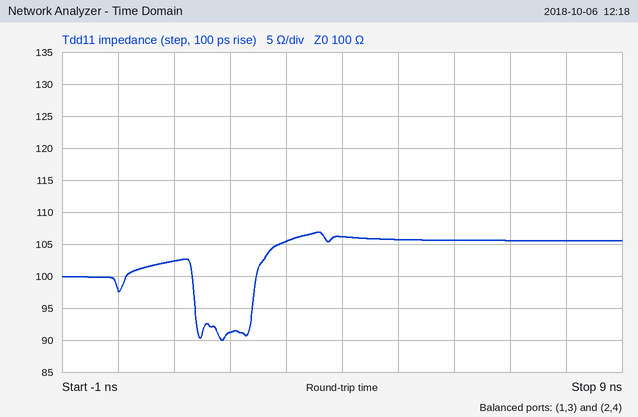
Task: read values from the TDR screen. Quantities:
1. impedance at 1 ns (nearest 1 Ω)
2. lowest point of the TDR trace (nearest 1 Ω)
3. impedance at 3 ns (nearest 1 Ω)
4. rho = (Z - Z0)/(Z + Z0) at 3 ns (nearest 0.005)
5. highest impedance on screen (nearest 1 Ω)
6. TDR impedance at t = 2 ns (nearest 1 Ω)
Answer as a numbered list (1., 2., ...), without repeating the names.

1. 102 Ω
2. 90 Ω
3. 105 Ω
4. +0.025
5. 107 Ω
6. 91 Ω
